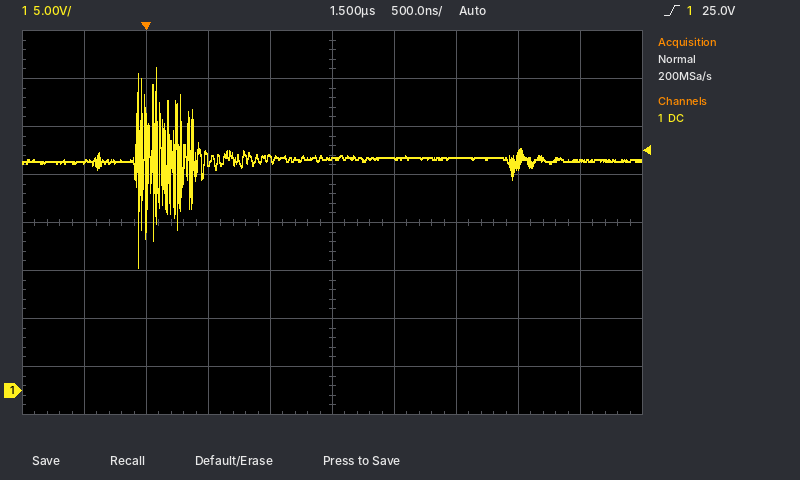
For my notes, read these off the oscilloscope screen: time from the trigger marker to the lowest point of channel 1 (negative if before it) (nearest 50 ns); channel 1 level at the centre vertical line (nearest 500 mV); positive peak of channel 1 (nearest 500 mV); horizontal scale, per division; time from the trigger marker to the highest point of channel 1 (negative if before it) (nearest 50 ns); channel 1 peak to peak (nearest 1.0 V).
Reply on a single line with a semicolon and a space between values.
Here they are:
-50 ns; 24.0 V; 33.5 V; 500 ns; +100 ns; 21.0 V
